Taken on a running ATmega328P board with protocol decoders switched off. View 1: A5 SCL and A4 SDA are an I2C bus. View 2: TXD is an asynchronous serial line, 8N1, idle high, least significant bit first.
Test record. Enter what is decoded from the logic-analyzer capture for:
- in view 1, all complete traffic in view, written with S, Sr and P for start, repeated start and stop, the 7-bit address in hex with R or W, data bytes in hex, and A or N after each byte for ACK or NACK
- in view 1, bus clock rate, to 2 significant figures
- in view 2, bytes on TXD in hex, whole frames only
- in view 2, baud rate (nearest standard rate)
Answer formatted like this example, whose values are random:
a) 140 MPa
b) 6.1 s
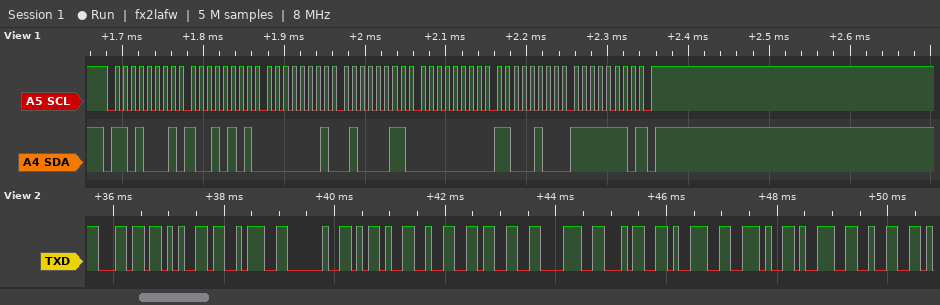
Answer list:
a) S 68R A 95 A 01 A 43 A 00 A C4 A FE N P
b) 100 kHz
c) 6C 65 3A 20 2D 32 33 38 34 39 2E 39 32
d) 9600 baud
